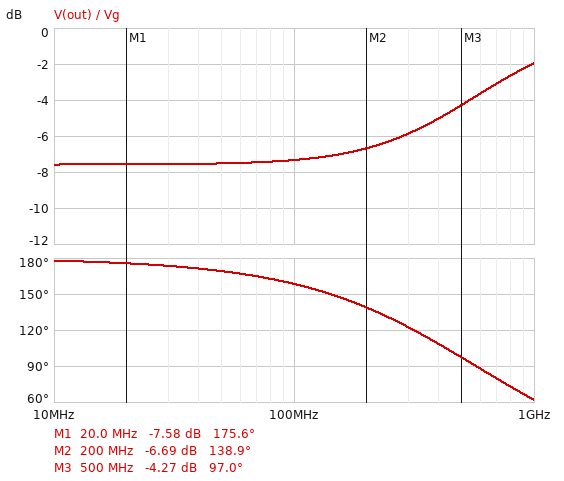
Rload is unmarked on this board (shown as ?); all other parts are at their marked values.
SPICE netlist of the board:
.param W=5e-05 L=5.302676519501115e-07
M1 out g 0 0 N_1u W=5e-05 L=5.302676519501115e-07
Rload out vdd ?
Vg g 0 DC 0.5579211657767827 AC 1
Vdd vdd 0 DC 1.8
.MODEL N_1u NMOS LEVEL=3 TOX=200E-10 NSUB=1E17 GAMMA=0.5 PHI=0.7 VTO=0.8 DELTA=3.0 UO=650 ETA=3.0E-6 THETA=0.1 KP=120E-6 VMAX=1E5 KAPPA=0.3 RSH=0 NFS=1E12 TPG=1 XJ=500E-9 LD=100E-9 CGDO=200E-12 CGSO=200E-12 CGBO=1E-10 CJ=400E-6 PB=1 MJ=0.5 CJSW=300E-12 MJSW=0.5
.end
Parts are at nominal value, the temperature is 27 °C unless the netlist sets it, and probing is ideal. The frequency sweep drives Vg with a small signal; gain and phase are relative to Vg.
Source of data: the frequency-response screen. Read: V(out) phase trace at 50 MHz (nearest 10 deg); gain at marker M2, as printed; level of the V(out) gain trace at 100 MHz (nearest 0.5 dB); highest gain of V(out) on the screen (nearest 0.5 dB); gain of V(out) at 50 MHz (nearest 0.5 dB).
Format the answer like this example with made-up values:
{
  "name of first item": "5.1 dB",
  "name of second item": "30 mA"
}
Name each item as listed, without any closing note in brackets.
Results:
{
  "V(out) phase trace at 50 MHz": "170 deg",
  "gain at marker M2, as printed": "-6.69 dB",
  "level of the V(out) gain trace at 100 MHz": "-7.5 dB",
  "highest gain of V(out) on the screen": "-2.0 dB",
  "gain of V(out) at 50 MHz": "-7.5 dB"
}
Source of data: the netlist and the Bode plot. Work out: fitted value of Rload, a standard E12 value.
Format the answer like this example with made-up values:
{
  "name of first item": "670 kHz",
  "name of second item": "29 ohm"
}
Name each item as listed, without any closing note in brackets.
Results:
{
  "fitted value of Rload, a standard E12 value": "18 kΩ"
}
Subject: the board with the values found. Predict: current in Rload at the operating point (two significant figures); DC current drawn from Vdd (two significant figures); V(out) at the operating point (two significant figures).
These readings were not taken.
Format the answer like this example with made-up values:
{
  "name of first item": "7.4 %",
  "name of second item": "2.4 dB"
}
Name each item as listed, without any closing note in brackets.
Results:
{
  "current in Rload at the operating point": "1.3 µA",
  "DC current drawn from Vdd": "1.3 µA",
  "V(out) at the operating point": "1.8 V"
}
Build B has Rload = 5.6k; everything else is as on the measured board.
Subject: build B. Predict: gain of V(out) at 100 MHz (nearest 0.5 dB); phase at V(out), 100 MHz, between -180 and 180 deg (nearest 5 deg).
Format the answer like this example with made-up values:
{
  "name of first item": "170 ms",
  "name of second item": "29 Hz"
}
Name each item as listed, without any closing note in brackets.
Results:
{
  "gain of V(out) at 100 MHz": "-17.5 dB",
  "phase at V(out), 100 MHz, between -180 and 180 deg": "165 deg"
}
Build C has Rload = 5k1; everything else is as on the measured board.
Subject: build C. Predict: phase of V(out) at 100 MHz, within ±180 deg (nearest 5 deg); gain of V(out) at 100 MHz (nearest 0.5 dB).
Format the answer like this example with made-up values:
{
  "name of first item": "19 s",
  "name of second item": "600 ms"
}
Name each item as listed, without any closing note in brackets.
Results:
{
  "phase of V(out) at 100 MHz, within ±180 deg": "165 deg",
  "gain of V(out) at 100 MHz": "-18.0 dB"
}
